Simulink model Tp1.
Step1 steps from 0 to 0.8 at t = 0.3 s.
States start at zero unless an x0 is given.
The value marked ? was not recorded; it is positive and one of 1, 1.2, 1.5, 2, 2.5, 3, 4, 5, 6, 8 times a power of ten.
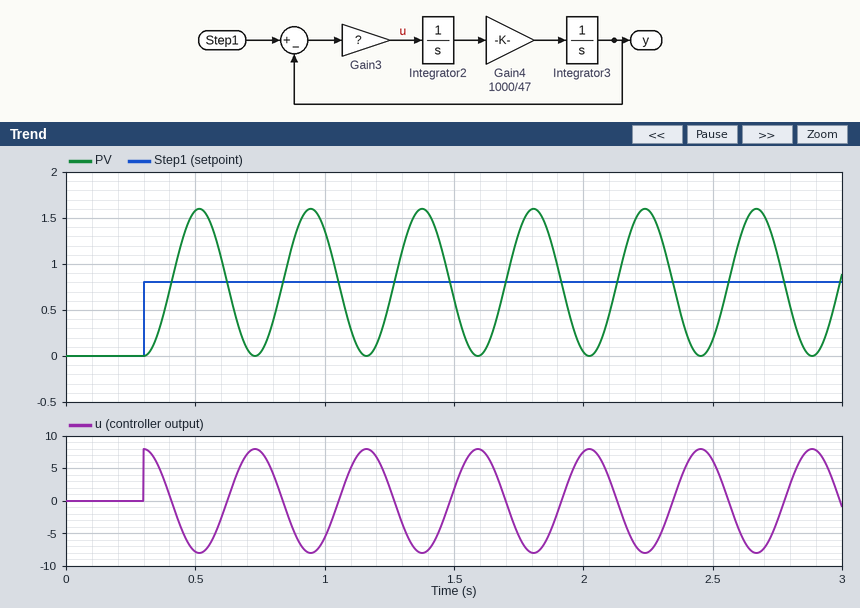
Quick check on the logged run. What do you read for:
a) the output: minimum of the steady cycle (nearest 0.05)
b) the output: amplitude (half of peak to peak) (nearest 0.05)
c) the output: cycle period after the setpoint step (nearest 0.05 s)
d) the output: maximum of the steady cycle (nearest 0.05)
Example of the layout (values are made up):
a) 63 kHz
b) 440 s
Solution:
a) 0.00
b) 0.80
c) 0.45 s
d) 1.60
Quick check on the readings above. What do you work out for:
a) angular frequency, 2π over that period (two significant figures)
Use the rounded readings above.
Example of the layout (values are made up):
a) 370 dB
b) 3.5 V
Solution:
a) 14 rad/s
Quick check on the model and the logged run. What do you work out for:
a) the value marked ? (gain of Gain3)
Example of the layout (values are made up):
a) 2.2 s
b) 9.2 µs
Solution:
a) 10
